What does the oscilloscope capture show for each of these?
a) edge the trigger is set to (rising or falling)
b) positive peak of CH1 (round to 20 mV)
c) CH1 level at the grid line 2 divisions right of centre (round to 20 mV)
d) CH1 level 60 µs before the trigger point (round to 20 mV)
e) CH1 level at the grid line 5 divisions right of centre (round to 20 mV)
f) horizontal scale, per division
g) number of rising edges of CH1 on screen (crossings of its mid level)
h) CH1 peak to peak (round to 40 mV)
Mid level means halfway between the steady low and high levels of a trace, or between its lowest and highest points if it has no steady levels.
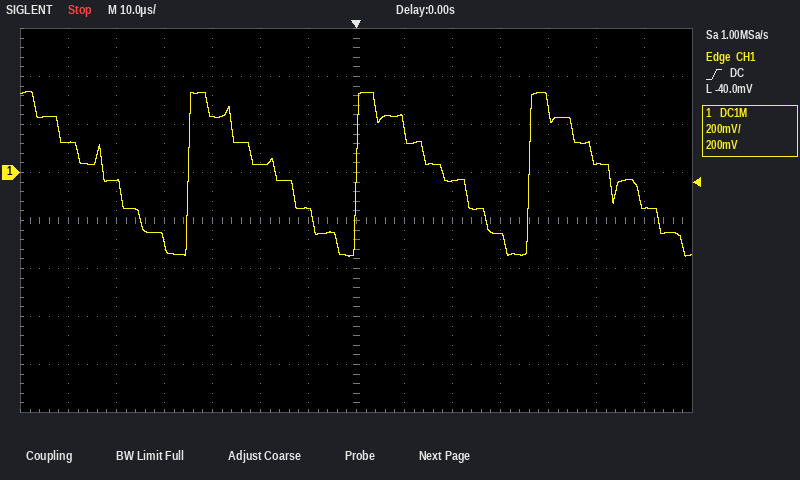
rising
340 mV
-40 mV
120 mV
40 mV
10 µs
3
680 mV
